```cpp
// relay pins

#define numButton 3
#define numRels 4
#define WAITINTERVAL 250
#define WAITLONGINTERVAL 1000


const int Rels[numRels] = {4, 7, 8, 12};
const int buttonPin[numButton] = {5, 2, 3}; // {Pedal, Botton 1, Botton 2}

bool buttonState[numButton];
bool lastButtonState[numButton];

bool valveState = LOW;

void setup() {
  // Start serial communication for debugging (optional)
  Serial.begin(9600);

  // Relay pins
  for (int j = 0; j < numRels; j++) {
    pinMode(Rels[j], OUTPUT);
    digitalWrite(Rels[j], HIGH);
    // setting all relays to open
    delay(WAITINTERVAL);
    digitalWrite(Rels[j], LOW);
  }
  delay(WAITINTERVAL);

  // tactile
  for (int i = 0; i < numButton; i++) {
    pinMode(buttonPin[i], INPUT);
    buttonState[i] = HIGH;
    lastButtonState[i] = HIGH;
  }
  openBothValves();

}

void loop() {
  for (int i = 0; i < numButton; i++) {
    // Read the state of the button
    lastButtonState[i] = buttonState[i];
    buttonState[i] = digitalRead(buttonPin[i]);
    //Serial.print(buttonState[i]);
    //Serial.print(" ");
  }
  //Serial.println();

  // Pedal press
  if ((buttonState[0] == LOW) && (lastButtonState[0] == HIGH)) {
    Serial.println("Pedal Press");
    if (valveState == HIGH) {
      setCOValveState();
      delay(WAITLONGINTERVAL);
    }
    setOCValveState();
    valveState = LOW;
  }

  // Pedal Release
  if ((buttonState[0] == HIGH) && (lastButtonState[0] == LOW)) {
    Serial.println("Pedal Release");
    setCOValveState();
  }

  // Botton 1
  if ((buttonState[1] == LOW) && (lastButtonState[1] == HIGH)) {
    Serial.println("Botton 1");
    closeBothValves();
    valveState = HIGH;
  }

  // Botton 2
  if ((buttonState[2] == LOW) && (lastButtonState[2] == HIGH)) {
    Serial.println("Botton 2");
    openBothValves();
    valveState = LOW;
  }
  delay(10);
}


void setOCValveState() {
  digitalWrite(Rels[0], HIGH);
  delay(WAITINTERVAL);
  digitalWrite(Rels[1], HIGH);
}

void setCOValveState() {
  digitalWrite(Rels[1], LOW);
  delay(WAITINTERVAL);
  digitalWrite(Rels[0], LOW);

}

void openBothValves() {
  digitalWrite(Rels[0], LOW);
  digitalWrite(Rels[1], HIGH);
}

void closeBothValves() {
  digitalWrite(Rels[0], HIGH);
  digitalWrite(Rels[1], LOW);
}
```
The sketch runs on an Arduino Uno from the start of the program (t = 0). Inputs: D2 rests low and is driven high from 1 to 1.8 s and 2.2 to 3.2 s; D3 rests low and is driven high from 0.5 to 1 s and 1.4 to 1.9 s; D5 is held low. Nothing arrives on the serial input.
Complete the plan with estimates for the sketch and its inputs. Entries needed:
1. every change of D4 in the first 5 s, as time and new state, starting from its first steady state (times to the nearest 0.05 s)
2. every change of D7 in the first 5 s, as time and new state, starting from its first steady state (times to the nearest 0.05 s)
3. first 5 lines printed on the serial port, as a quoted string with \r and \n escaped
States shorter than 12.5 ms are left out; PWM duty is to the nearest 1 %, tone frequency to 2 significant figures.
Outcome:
0 s high; 0.25 s low; 1.25 s high; 1.5 s low; 1.8 s high; 1.9 s low; 3.2 s high
0.25 s high; 0.5 s low; 1.25 s high; 1.8 s low; 1.9 s high; 3.2 s low
"Pedal Press\r\nBotton 2\r\nBotton 1\r\nBotton 2\r\nBotton 1\r\n"
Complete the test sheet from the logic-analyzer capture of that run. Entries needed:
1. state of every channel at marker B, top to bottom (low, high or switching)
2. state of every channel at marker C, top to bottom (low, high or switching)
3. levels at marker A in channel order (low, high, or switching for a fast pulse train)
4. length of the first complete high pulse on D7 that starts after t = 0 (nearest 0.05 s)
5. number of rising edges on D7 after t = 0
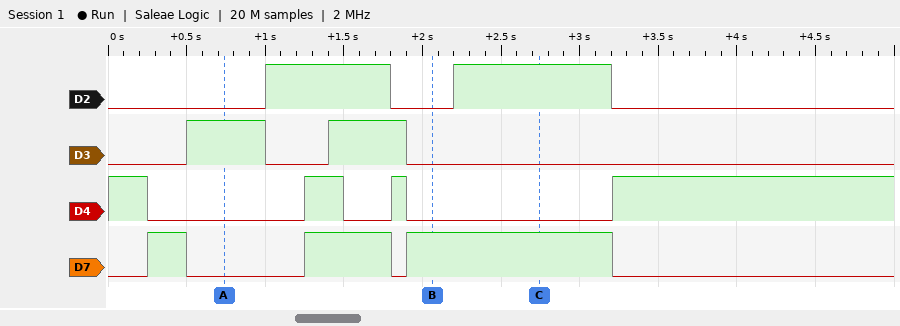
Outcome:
D2 low, D3 low, D4 low, D7 high
D2 high, D3 low, D4 low, D7 high
D2 low, D3 high, D4 low, D7 low
0.25 s
3
